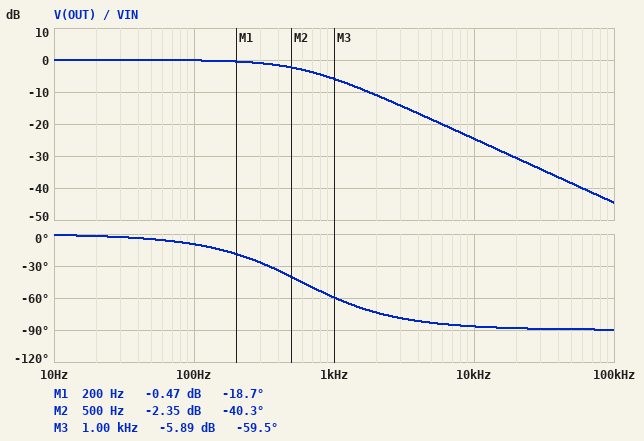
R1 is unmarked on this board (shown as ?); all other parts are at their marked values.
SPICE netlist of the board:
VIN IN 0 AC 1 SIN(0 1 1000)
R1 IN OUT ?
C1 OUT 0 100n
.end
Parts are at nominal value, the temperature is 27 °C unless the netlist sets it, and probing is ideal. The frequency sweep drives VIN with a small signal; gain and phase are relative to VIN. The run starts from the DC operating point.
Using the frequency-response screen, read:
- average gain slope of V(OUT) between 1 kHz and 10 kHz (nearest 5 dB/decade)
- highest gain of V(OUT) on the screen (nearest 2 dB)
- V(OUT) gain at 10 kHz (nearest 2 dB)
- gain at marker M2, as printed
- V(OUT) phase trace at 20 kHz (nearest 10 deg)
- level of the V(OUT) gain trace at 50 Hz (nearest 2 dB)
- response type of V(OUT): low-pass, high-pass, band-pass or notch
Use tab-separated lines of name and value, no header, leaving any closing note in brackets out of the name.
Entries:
average gain slope of V(OUT) between 1 kHz and 10 kHz	-20 dB/decade
highest gain of V(OUT) on the screen	0 dB
V(OUT) gain at 10 kHz	-24 dB
gain at marker M2, as printed	-2.35 dB
V(OUT) phase trace at 20 kHz	-90 deg
level of the V(OUT) gain trace at 50 Hz	0 dB
response type of V(OUT): low-pass, high-pass, band-pass or notch	low-pass
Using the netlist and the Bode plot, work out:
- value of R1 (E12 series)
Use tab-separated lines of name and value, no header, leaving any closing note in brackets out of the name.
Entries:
value of R1	2.7 kΩ
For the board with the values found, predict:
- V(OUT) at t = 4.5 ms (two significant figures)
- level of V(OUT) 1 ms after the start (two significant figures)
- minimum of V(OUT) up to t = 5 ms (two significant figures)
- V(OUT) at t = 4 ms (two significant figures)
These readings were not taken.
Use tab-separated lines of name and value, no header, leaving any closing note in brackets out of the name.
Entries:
V(OUT) at t = 4.5 ms	440 mV
level of V(OUT) 1 ms after the start	-430 mV
minimum of V(OUT) up to t = 5 ms	-510 mV
V(OUT) at t = 4 ms	-440 mV
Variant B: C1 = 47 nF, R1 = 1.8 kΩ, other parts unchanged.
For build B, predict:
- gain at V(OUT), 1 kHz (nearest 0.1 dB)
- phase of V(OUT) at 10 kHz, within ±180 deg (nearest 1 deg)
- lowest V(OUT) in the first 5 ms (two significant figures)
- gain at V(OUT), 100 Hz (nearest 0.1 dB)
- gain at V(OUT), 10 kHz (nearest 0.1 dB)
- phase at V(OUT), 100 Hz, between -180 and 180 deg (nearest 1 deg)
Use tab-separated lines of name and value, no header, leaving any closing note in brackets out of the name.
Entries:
gain at V(OUT), 1 kHz	-1.1 dB
phase of V(OUT) at 10 kHz, within ±180 deg	-79 deg
lowest V(OUT) in the first 5 ms	-880 mV
gain at V(OUT), 100 Hz	0 dB
gain at V(OUT), 10 kHz	-14.7 dB
phase at V(OUT), 100 Hz, between -180 and 180 deg	-3 deg
